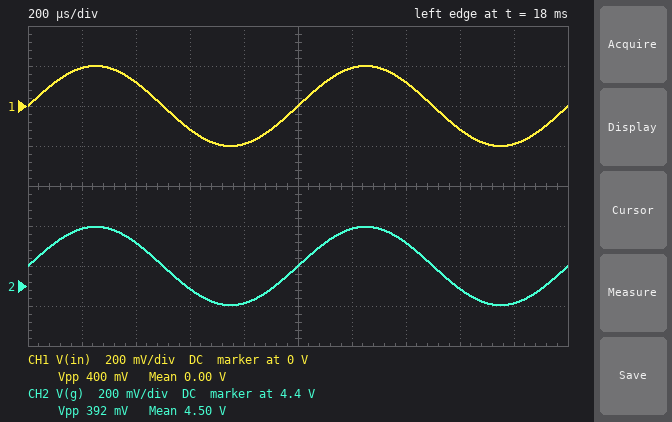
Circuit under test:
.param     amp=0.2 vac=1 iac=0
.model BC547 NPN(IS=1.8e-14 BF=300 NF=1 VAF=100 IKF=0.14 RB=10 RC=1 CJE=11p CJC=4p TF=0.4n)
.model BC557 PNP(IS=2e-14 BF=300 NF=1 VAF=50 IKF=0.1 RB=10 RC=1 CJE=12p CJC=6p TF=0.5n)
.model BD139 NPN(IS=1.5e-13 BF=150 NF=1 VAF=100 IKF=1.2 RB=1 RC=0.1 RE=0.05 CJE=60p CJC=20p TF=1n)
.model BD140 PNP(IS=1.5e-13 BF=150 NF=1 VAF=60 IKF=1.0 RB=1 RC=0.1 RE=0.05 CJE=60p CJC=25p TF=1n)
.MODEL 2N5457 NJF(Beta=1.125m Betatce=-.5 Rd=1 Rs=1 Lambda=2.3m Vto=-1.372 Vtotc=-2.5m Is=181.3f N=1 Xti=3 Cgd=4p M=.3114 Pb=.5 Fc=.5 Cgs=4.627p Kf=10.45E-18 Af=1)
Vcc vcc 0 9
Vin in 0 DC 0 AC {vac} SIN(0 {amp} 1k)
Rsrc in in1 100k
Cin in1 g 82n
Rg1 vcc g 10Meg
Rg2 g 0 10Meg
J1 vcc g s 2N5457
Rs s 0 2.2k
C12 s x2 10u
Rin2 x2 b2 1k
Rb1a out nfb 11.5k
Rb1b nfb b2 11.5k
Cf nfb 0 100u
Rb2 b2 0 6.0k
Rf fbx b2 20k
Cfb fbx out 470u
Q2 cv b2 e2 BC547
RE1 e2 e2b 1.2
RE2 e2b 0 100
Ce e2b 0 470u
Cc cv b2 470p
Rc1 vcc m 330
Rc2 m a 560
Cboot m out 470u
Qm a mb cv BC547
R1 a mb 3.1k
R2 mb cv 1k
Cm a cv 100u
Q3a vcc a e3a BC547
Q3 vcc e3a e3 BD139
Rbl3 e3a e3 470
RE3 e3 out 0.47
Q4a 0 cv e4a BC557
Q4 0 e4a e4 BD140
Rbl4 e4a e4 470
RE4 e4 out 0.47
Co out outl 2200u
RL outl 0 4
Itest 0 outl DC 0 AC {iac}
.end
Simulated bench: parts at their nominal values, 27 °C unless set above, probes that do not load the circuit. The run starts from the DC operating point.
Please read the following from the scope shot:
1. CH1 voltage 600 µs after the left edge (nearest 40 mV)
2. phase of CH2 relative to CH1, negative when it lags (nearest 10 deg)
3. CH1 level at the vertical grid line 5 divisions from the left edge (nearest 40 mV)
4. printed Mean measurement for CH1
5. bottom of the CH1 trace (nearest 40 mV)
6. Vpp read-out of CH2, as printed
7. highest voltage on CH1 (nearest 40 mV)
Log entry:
-120 mV
0 deg
0 V
0.00 V
-200 mV
392 mV
200 mV
